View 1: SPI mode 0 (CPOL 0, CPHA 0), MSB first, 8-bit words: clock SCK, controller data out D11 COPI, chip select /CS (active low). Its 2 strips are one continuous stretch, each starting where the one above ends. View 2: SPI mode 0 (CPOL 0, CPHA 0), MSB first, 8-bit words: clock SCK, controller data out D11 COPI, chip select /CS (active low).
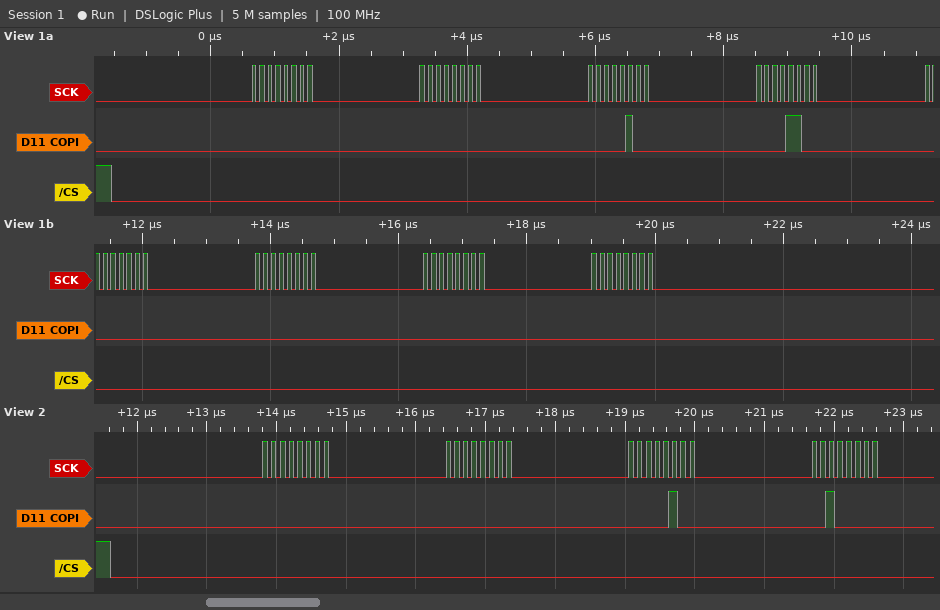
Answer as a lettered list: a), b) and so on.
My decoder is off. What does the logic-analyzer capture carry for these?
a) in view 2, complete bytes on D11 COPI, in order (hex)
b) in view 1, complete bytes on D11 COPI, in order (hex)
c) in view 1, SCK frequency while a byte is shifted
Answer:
a) 00 00 04 20
b) 00 00 04 0C 00 00 00 00
c) 8 MHz
